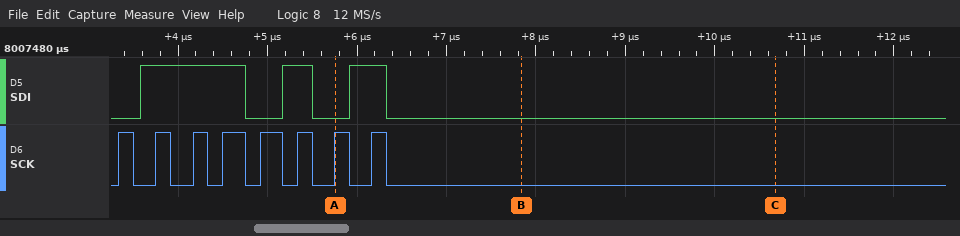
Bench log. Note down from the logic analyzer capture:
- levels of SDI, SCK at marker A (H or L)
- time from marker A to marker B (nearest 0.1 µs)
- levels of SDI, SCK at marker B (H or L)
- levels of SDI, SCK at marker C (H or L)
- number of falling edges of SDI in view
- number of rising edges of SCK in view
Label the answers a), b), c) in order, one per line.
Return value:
a) SDI=L, SCK=H
b) 2.1 µs
c) SDI=L, SCK=L
d) SDI=L, SCK=L
e) 3
f) 8
